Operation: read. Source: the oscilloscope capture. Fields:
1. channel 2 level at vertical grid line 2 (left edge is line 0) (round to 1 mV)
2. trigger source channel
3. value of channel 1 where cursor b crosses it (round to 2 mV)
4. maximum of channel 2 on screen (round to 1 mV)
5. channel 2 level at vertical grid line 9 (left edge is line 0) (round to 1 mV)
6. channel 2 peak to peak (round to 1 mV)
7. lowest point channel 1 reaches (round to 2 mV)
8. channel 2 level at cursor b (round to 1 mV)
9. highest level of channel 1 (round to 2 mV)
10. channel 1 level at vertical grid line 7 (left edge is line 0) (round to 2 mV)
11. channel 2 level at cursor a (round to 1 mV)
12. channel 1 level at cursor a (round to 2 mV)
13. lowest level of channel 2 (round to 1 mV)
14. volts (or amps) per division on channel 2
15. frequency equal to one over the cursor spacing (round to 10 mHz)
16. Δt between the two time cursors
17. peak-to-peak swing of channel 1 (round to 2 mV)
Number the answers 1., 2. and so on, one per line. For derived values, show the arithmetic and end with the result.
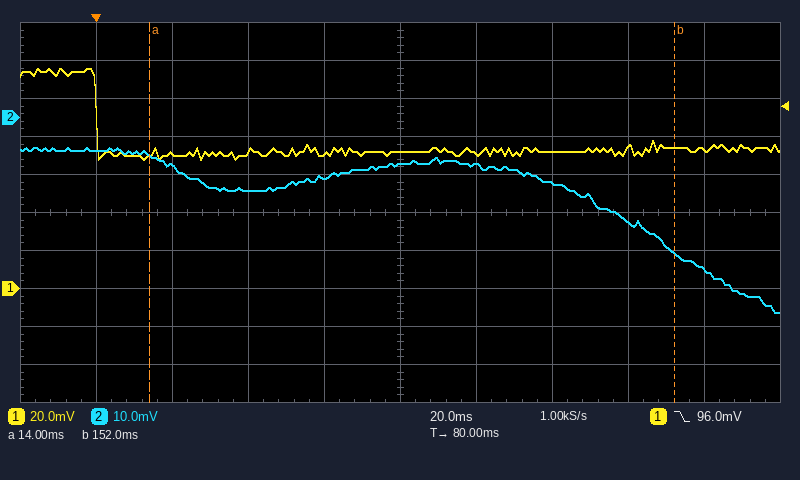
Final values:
1. -13 mV
2. channel 1
3. 74 mV
4. -8 mV
5. -40 mV
6. -8 mV − (-51 mV) = 43 mV
7. 68 mV
8. -36 mV
9. 116 mV
10. 72 mV
11. -10 mV
12. 70 mV
13. -51 mV
14. 10 mV
15. 1 / 138 ms ≈ 7.25 Hz
16. 152 ms − (14 ms) = 138 ms
17. 116 mV − (68 mV) = 48 mV
